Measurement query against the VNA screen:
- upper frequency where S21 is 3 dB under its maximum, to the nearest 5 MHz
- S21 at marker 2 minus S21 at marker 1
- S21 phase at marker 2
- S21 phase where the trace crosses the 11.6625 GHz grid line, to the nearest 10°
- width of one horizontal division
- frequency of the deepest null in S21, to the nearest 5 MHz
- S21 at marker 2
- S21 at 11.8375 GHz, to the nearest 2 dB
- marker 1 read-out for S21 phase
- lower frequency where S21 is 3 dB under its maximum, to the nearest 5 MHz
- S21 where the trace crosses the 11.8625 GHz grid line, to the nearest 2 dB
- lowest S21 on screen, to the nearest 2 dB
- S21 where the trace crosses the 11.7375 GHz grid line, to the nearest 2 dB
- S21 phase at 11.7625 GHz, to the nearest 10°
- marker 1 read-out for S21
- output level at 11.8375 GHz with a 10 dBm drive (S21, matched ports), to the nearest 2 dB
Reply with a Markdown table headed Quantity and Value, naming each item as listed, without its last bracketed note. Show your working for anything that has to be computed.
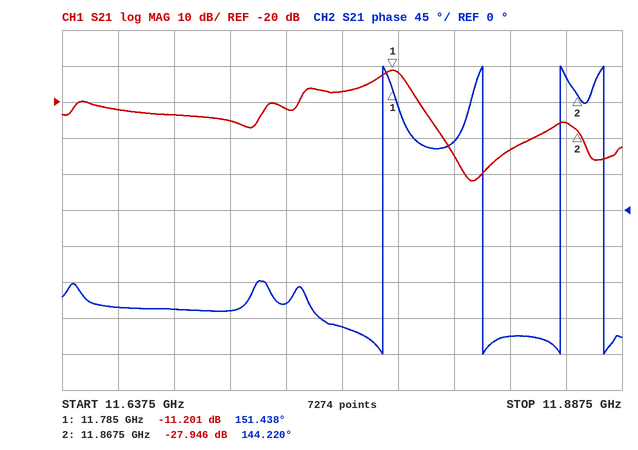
| Quantity | Value |
|---|---|
| upper frequency where S21 is 3 dB under its maximum, to the nearest 5 MHz | 11.790 GHz |
| S21 at marker 2 minus S21 at marker 1 | -27.946 − (-11.201) = -16.745 dB |
| S21 phase at marker 2 | 144.220° |
| S21 phase where the trace crosses the 11.6625 GHz grid line, to the nearest 10° | -120° |
| width of one horizontal division | 25 MHz |
| frequency of the deepest null in S21, to the nearest 5 MHz | 11.820 GHz |
| S21 at marker 2 | -27.946 dB |
| S21 at 11.8375 GHz, to the nearest 2 dB | -34 dB |
| marker 1 read-out for S21 phase | 151.438° |
| lower frequency where S21 is 3 dB under its maximum, to the nearest 5 MHz | 11.775 GHz |
| S21 where the trace crosses the 11.8625 GHz grid line, to the nearest 2 dB | -26 dB |
| lowest S21 on screen, to the nearest 2 dB | -42 dB |
| S21 where the trace crosses the 11.7375 GHz grid line, to the nearest 2 dB | -22 dB |
| S21 phase at 11.7625 GHz, to the nearest 10° | -150° |
| marker 1 read-out for S21 | -11.201 dB |
| output level at 11.8375 GHz with a 10 dBm drive (S21, matched ports), to the nearest 2 dB | 10 dBm + (-34 dB) = -24 dBm |
